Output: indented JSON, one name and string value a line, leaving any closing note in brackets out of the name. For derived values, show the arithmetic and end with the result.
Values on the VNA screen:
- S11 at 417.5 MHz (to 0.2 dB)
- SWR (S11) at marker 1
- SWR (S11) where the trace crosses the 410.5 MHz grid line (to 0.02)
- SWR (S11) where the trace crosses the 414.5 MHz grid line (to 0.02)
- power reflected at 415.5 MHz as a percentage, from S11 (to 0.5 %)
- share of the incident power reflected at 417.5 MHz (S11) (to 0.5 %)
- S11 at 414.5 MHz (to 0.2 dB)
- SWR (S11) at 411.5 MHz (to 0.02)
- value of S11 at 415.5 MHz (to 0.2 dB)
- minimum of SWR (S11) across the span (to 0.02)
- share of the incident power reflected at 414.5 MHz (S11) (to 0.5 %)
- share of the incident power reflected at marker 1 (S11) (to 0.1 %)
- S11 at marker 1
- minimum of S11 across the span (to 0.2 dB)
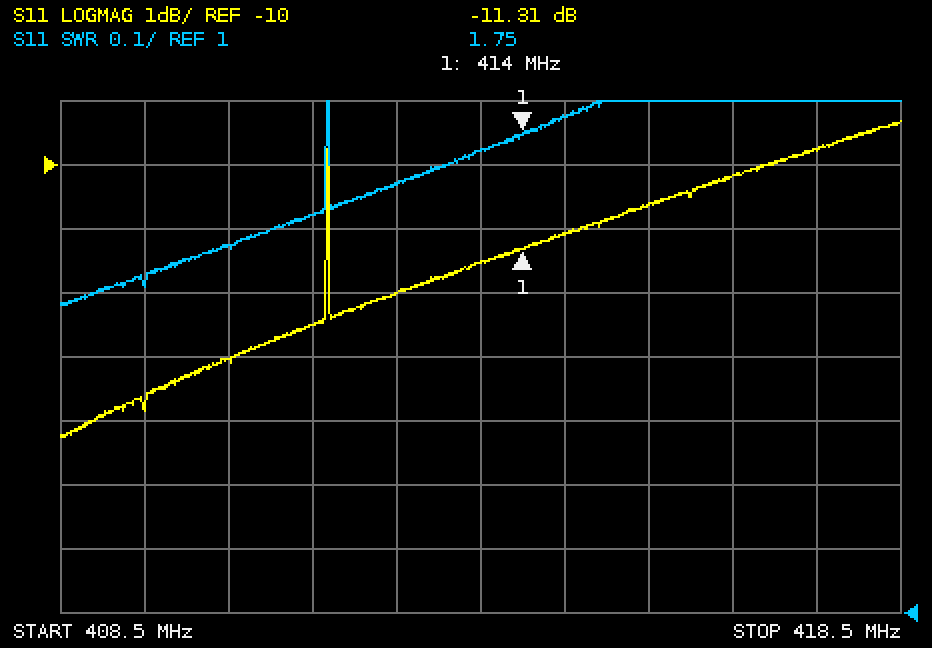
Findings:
{
  "S11 at 417.5 MHz": "-9.8 dB",
  "SWR (S11) at marker 1": "1.75",
  "SWR (S11) where the trace crosses the 410.5 MHz grid line": "1.58",
  "SWR (S11) where the trace crosses the 414.5 MHz grid line": "1.78",
  "power reflected at 415.5 MHz as a percentage, from S11": "10^(-10.6/10) ≈ 8.71 %, so 8.5 % to the nearest 0.5 %",
  "share of the incident power reflected at 417.5 MHz (S11)": "10^(-9.8/10) ≈ 10.5 %",
  "S11 at 414.5 MHz": "-11.0 dB",
  "SWR (S11) at 411.5 MHz": "1.62",
  "value of S11 at 415.5 MHz": "-10.6 dB",
  "minimum of SWR (S11) across the span": "1.48",
  "share of the incident power reflected at 414.5 MHz (S11)": "10^(-11/10) ≈ 7.94 %, so 8.0 % to the nearest 0.5 %",
  "share of the incident power reflected at marker 1 (S11)": "10^(-11.31/10) ≈ 7.4 %",
  "S11 at marker 1": "-11.31 dB",
  "minimum of S11 across the span": "-14.2 dB"
}
